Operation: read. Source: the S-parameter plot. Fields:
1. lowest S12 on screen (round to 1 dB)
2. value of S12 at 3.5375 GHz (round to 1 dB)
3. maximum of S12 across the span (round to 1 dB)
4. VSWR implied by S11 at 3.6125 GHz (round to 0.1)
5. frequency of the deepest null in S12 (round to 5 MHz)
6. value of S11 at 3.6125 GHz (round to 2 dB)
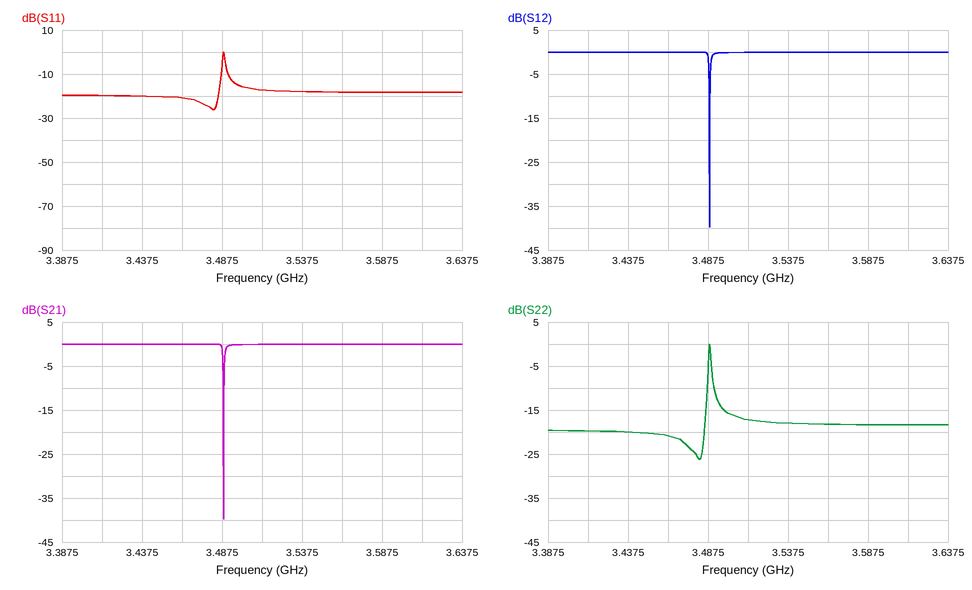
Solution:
-40 dB
0 dB
0 dB
1.3
3.490 GHz
-18 dB
